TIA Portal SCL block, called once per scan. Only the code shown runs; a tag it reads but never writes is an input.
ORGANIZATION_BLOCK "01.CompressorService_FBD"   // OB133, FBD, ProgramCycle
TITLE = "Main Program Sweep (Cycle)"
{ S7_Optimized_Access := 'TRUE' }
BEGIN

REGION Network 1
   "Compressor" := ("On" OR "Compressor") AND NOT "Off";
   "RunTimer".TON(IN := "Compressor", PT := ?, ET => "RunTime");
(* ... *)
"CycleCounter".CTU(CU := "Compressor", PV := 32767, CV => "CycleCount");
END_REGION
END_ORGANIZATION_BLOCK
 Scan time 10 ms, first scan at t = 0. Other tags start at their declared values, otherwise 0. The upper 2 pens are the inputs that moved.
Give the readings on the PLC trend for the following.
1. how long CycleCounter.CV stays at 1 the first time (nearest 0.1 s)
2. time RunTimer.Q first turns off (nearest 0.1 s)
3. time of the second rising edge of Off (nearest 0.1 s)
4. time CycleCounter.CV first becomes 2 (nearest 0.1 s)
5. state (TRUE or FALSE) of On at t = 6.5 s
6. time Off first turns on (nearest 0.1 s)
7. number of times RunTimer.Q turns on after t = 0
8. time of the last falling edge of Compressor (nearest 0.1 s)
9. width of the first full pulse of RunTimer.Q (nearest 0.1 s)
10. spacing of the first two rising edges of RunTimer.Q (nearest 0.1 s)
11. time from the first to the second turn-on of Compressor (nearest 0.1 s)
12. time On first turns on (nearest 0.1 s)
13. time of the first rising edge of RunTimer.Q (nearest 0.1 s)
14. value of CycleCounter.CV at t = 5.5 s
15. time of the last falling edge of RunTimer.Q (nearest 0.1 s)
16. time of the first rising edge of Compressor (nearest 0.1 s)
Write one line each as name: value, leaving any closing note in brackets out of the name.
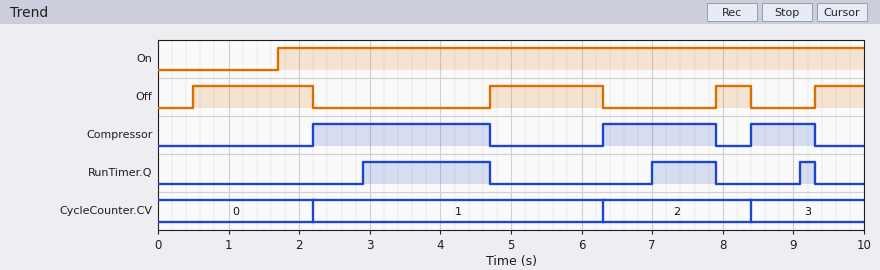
how long CycleCounter.CV stays at 1 the first time: 4.1 s
time RunTimer.Q first turns off: 4.7 s
time of the second rising edge of Off: 4.7 s
time CycleCounter.CV first becomes 2: 6.3 s
state (TRUE or FALSE) of On at t = 6.5 s: TRUE
time Off first turns on: 0.5 s
number of times RunTimer.Q turns on after t = 0: 3
time of the last falling edge of Compressor: 9.3 s
width of the first full pulse of RunTimer.Q: 1.8 s
spacing of the first two rising edges of RunTimer.Q: 4.1 s
time from the first to the second turn-on of Compressor: 4.1 s
time On first turns on: 1.7 s
time of the first rising edge of RunTimer.Q: 2.9 s
value of CycleCounter.CV at t = 5.5 s: 1
time of the last falling edge of RunTimer.Q: 9.3 s
time of the first rising edge of Compressor: 2.2 s
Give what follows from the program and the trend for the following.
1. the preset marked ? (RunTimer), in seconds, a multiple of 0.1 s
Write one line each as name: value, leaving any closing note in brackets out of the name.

the preset marked ? (RunTimer), in seconds, a multiple of 0.1 s: 0.7 s
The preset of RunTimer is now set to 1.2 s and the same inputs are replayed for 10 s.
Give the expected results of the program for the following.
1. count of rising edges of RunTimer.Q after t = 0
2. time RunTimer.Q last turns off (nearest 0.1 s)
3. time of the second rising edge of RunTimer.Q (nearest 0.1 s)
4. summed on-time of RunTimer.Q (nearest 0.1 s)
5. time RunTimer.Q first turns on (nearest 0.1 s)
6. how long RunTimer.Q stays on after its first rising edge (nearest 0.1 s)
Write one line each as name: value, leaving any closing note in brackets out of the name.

count of rising edges of RunTimer.Q after t = 0: 2
time RunTimer.Q last turns off: 7.9 s
time of the second rising edge of RunTimer.Q: 7.5 s
summed on-time of RunTimer.Q: 1.7 s
time RunTimer.Q first turns on: 3.4 s
how long RunTimer.Q stays on after its first rising edge: 1.3 s
